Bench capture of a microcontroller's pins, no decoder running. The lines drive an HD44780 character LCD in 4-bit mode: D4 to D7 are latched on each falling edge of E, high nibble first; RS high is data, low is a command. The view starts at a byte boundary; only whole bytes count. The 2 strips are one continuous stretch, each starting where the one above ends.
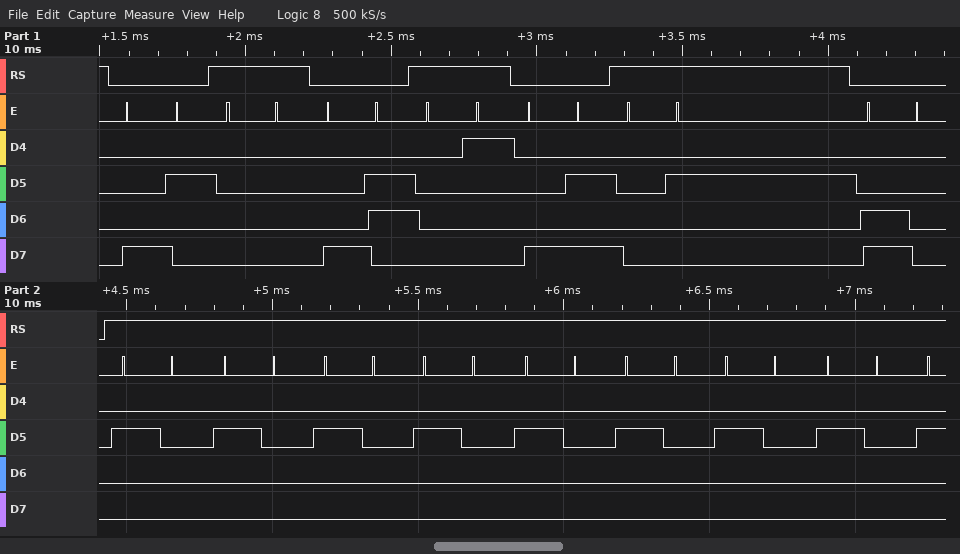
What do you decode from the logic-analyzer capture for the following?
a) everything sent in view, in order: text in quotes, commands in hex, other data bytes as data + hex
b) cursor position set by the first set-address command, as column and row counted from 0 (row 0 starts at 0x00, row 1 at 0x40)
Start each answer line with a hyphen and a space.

- 0x82 data 00 0x86 data 01 0x8A data 02 0xC0 "        "
- column 2, row 0
